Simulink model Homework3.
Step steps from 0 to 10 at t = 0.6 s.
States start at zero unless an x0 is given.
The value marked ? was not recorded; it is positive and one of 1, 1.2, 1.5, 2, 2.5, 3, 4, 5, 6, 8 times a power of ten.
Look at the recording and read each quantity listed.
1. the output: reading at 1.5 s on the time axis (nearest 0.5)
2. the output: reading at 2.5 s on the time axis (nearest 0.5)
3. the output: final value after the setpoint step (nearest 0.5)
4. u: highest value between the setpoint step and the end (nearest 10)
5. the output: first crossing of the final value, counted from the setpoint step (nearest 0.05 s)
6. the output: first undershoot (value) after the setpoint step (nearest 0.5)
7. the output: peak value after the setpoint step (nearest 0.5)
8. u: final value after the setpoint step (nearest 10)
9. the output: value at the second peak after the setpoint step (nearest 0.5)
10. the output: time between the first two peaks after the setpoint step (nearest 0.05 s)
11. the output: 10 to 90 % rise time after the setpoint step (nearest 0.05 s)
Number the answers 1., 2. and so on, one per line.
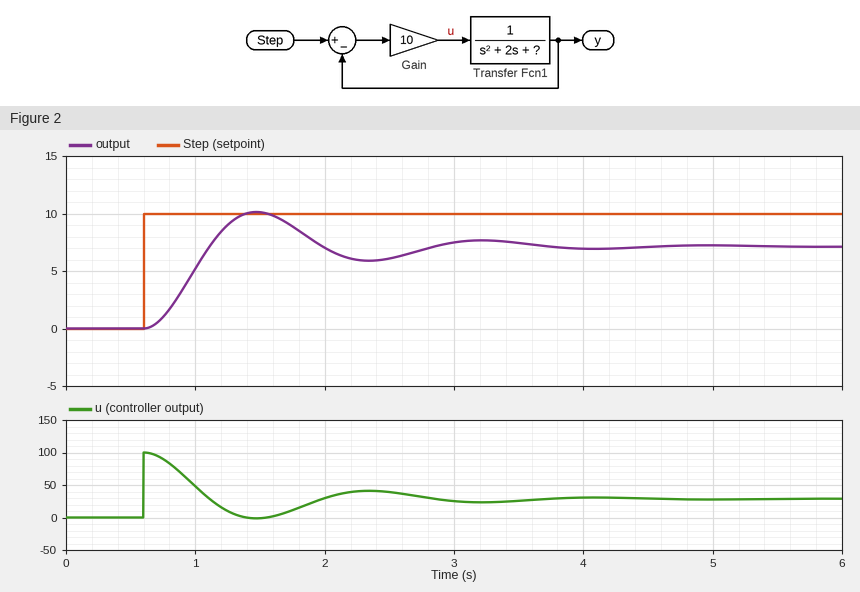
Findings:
1. 10.0
2. 6.0
3. 7.0
4. 100
5. 0.50 s
6. 6.0
7. 10.0
8. 30
9. 7.5
10. 1.75 s
11. 0.35 s
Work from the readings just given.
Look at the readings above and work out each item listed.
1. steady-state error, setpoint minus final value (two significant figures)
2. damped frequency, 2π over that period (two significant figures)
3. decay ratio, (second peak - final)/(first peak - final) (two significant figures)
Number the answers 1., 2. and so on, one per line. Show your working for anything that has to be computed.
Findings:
1. 10 - 7 = 3.0
2. 2π / 1.75 = 3.6 rad/s
3. (7.5 - 7) / (10 - 7) = 0.17
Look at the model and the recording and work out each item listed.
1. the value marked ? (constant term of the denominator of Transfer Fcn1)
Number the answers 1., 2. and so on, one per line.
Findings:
1. 4
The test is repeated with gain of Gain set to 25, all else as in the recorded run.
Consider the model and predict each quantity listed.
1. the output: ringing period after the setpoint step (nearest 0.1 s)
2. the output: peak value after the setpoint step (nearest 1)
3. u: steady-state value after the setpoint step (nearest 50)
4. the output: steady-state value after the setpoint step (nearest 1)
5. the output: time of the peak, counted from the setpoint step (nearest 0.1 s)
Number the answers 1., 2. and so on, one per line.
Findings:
1. 1.2 s
2. 13
3. 50
4. 9
5. 0.6 s
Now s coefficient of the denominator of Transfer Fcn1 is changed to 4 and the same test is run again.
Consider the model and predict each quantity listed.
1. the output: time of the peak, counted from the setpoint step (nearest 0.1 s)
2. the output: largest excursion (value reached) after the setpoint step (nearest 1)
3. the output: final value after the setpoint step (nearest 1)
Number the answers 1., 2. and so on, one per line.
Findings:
1. 1.0 s
2. 8
3. 7
